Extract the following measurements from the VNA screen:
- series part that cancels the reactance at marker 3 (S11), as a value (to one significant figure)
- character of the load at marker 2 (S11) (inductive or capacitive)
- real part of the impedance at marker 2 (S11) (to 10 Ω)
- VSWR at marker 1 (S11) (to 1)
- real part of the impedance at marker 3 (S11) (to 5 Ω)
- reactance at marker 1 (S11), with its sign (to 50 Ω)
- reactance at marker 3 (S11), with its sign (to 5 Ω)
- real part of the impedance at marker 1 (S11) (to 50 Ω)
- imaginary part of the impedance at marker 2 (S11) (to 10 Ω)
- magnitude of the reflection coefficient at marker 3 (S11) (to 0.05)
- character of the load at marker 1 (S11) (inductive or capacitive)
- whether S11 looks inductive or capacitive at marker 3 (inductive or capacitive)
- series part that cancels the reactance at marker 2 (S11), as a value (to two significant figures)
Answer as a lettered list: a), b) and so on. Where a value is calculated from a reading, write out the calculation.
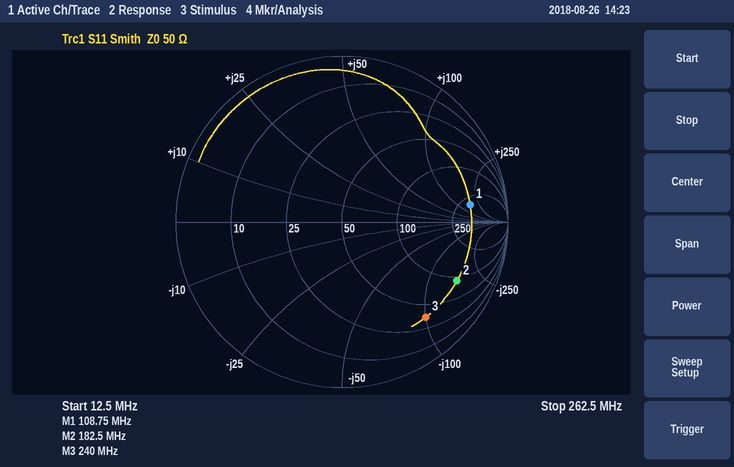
a) L = 100 Ω/(2π × 240 MHz) ≈ 66.3 nH, so 70 nH to one significant figure
b) capacitive
c) 90 Ω
d) 8
e) 35 Ω
f) +150 Ω
g) -100 Ω
h) 300 Ω
i) -160 Ω
j) 0.75
k) inductive
l) capacitive
m) L = 160 Ω/(2π × 182.5 MHz) ≈ 140 nH
